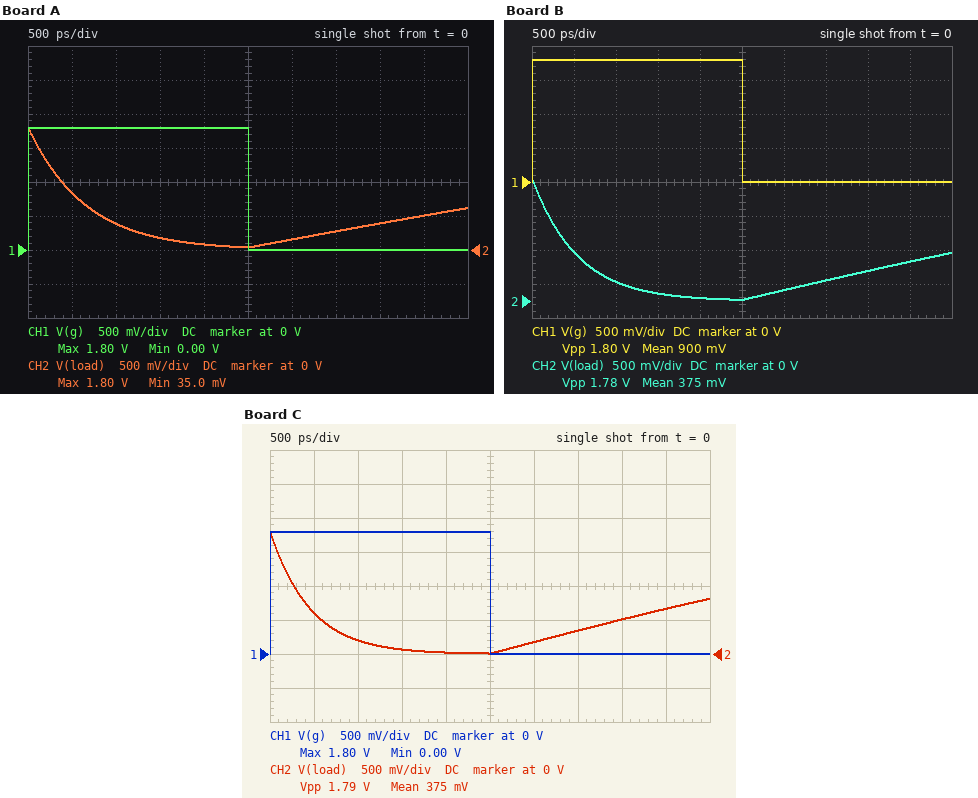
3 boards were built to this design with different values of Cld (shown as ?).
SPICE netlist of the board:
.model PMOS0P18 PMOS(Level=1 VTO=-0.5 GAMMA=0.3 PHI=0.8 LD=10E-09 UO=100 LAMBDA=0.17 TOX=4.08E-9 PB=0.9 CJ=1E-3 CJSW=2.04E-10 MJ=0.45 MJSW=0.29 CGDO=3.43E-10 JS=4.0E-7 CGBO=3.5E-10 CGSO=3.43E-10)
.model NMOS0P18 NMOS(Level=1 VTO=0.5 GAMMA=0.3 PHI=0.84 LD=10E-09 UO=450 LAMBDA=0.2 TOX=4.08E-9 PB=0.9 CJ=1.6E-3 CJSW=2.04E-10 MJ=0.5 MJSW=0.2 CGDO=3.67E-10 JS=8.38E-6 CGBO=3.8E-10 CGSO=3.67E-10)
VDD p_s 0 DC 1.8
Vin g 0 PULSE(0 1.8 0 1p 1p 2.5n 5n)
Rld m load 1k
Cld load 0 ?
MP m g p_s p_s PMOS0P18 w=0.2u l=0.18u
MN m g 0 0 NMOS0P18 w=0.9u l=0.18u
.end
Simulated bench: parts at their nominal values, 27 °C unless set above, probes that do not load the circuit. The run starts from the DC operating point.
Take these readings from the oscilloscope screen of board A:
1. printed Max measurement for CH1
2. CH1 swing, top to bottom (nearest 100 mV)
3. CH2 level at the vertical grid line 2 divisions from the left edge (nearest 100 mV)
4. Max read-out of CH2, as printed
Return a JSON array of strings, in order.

["1.80 V", "1.8 V", "400 mV", "1.80 V"]
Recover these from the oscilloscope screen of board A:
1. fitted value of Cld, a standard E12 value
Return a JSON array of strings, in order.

["470 fF"]
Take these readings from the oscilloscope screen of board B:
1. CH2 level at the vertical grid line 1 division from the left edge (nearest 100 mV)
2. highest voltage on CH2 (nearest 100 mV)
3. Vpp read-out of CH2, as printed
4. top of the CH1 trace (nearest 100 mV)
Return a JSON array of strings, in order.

["700 mV", "1.8 V", "1.78 V", "1.8 V"]
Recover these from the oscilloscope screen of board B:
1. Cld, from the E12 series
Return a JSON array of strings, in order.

["390 fF"]
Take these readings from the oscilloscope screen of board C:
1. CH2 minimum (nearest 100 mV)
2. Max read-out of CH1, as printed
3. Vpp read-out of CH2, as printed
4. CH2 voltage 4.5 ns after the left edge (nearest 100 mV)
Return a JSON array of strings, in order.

["0 V", "1.80 V", "1.79 V", "700 mV"]
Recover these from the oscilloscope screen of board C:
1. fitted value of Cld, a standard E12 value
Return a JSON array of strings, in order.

["330 fF"]
